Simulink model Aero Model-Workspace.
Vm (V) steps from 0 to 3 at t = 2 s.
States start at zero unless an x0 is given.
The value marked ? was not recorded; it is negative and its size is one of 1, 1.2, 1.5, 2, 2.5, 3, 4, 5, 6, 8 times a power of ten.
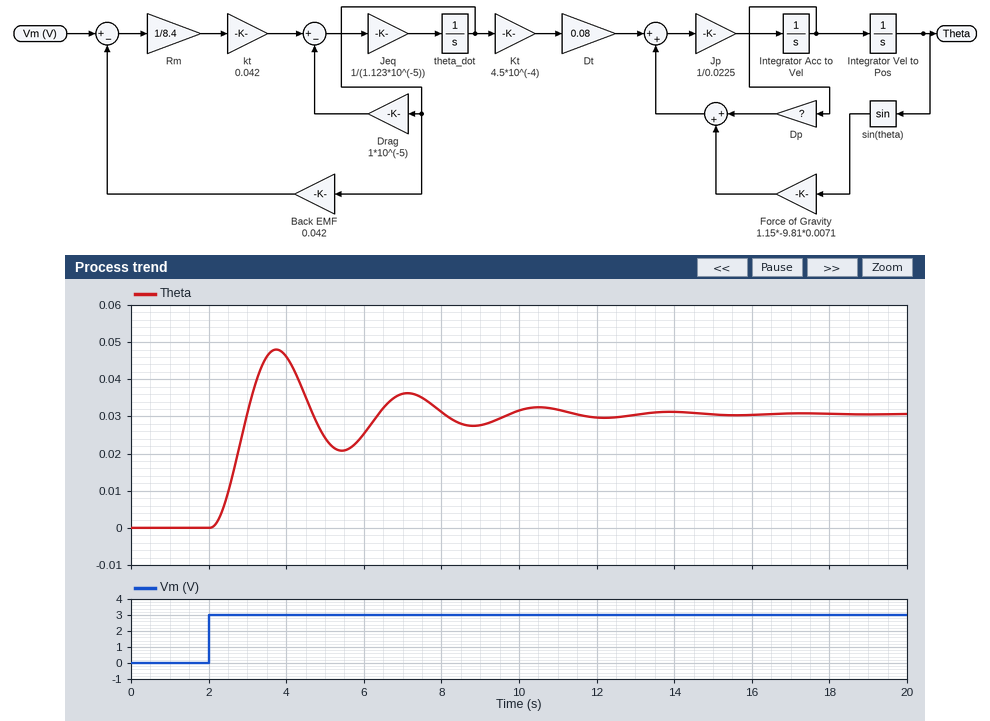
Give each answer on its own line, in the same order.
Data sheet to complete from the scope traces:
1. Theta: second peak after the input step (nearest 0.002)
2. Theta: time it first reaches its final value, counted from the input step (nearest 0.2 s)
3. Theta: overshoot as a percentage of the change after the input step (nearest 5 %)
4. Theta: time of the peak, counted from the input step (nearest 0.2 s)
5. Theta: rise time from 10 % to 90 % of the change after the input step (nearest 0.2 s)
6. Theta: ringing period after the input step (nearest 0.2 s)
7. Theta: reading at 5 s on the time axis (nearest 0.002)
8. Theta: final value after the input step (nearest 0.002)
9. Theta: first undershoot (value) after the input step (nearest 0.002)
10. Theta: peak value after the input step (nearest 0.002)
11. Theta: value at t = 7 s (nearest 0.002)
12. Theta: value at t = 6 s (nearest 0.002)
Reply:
0.036
1.0 s
55 %
1.8 s
0.6 s
3.4 s
0.024
0.030
0.020
0.048
0.036
0.026
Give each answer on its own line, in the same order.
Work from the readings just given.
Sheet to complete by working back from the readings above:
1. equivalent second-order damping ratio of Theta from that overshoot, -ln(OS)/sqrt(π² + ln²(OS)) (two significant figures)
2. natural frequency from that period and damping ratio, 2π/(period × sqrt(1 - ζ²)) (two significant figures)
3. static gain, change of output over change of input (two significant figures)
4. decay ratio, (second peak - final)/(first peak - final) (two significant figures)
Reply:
0.19
1.9 rad/s
0.010
0.33
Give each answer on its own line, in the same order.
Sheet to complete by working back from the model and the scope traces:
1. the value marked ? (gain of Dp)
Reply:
-0.015
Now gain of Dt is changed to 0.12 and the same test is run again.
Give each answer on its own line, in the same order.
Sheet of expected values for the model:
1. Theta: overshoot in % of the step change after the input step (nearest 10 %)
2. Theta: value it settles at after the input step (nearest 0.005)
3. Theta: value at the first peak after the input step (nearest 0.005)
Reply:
60 %
0.045
0.070
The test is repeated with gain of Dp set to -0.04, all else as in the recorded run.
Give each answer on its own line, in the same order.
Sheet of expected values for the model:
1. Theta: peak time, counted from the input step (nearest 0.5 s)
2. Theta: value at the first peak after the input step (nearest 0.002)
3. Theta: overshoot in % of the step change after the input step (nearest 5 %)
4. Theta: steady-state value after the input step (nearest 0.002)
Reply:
2.0 s
0.036
20 %
0.030
